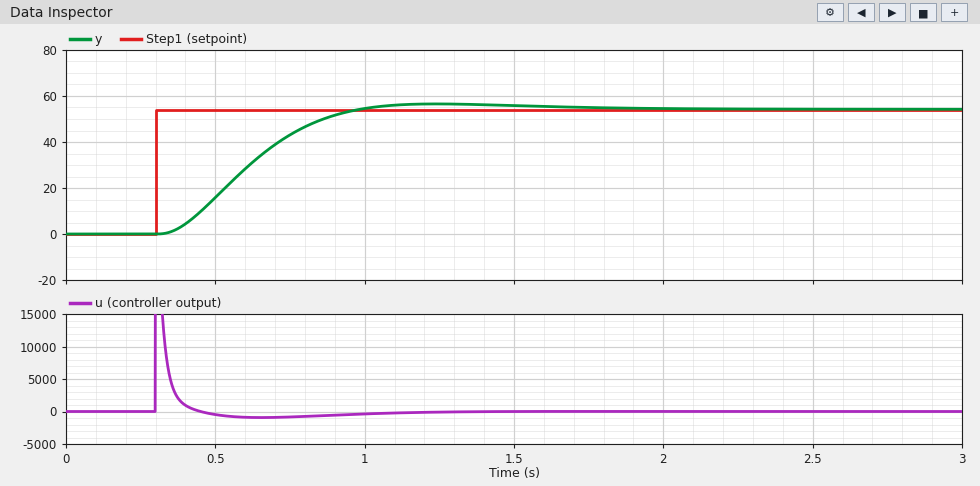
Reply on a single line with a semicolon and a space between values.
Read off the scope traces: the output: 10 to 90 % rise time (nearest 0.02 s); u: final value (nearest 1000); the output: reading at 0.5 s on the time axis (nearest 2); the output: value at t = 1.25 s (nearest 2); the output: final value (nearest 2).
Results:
0.42 s; 0; 16; 56; 54
